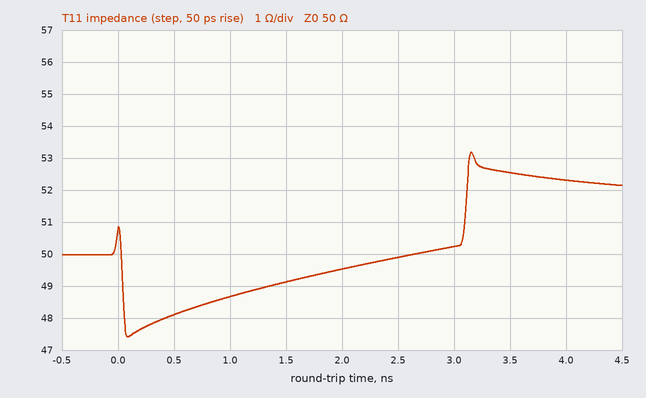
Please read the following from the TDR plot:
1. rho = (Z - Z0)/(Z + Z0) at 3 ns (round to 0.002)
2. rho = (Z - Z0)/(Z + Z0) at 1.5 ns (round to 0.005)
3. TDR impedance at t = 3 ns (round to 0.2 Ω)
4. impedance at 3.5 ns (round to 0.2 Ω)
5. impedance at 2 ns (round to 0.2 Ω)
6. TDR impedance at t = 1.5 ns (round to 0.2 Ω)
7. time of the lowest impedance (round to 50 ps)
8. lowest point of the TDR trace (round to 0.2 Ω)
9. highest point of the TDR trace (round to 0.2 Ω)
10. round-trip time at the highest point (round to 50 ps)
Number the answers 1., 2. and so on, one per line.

1. +0.002
2. -0.010
3. 50.2 Ω
4. 52.6 Ω
5. 49.6 Ω
6. 49.2 Ω
7. 100 ps
8. 47.4 Ω
9. 53.2 Ω
10. 3.15 ns
